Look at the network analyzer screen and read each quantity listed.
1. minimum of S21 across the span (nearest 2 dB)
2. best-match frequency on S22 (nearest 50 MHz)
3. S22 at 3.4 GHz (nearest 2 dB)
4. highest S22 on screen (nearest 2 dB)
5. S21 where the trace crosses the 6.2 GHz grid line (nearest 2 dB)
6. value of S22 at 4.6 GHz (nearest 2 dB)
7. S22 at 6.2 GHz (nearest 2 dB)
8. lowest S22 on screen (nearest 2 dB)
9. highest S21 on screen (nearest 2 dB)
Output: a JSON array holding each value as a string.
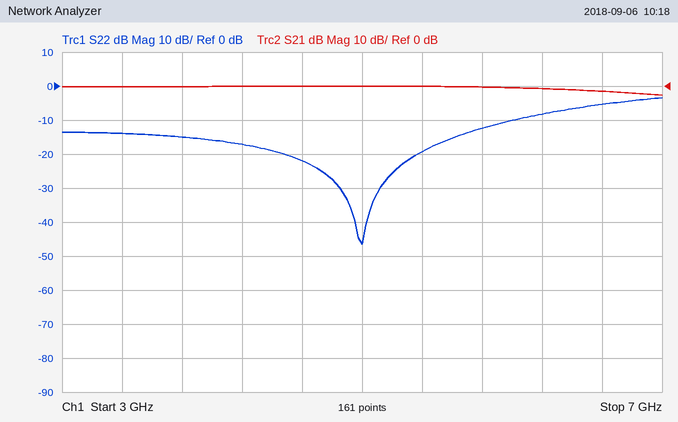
["-2 dB", "5.00 GHz", "-14 dB", "-4 dB", "0 dB", "-22 dB", "-8 dB", "-46 dB", "0 dB"]
